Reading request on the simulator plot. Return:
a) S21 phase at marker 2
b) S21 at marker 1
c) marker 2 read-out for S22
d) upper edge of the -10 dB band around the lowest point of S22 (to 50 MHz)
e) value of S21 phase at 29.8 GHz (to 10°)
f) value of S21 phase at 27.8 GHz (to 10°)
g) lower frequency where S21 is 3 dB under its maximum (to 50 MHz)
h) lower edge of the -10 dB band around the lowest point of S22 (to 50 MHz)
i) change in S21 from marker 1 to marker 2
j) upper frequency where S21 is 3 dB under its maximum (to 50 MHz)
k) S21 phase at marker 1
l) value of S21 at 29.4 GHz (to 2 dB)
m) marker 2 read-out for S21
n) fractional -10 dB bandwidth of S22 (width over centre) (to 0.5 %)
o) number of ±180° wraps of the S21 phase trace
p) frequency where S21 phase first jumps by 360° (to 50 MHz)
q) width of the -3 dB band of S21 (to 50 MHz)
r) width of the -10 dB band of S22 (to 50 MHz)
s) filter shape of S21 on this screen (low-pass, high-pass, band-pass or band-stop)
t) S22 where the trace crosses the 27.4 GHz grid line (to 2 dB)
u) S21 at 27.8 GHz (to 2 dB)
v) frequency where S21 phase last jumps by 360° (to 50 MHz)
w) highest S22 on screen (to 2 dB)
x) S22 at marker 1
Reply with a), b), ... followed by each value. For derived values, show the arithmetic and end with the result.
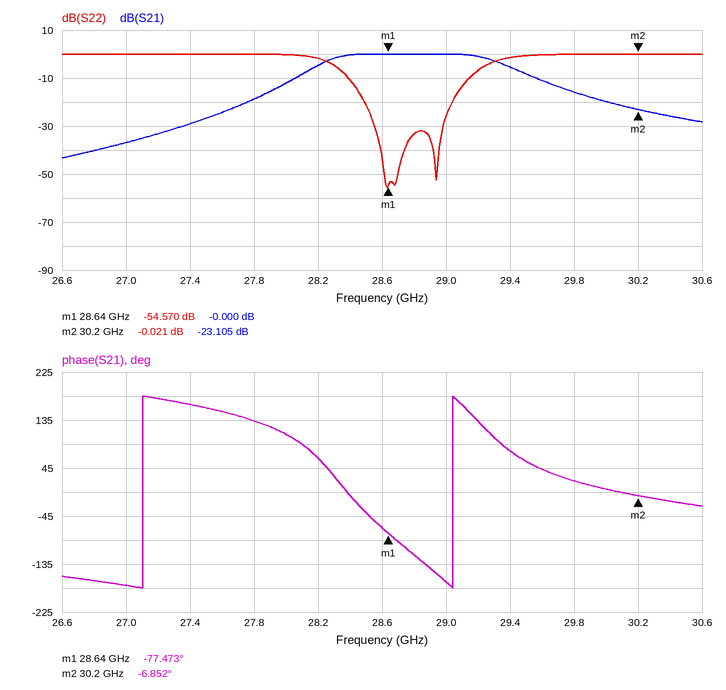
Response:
a) -6.852°
b) -0.000 dB
c) -0.021 dB
d) 29.15 GHz
e) 20°
f) 130°
g) 28.25 GHz
h) 28.40 GHz
i) -23.105 − (-0) = -23.105 dB
j) 29.30 GHz
k) -77.473°
l) -6 dB
m) -23.105 dB
n) 750 MHz / 28.775 GHz ≈ 2.61 %, so 2.5 % to the nearest 0.5 %
o) 2
p) 27.10 GHz
q) 29.30 GHz − 28.25 GHz = 1.05 GHz
r) 29.15 GHz − 28.40 GHz = 750 MHz
s) band-pass
t) 0 dB
u) -18 dB
v) 29.05 GHz
w) 0 dB
x) -54.570 dB
